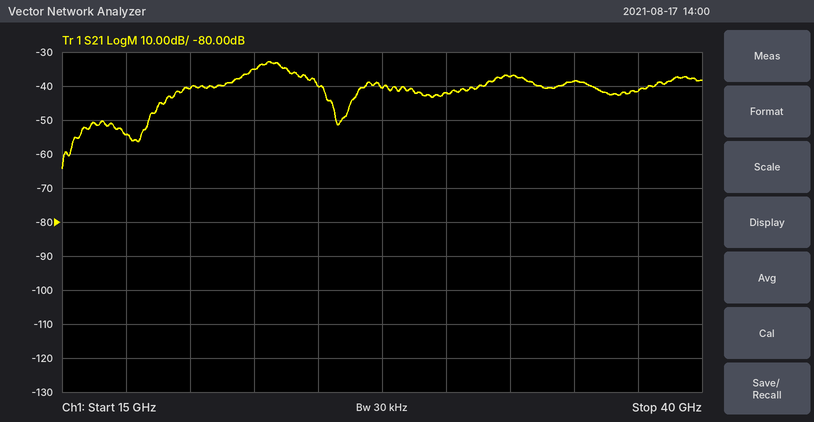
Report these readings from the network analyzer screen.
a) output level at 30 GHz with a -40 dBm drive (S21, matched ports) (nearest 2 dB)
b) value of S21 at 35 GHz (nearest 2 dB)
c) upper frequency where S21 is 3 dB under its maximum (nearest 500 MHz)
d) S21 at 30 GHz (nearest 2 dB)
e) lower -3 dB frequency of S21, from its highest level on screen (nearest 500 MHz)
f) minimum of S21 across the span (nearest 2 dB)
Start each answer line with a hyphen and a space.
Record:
- -82 dBm
- -38 dB
- 24.0 GHz
- -42 dB
- 22.5 GHz
- -64 dB
